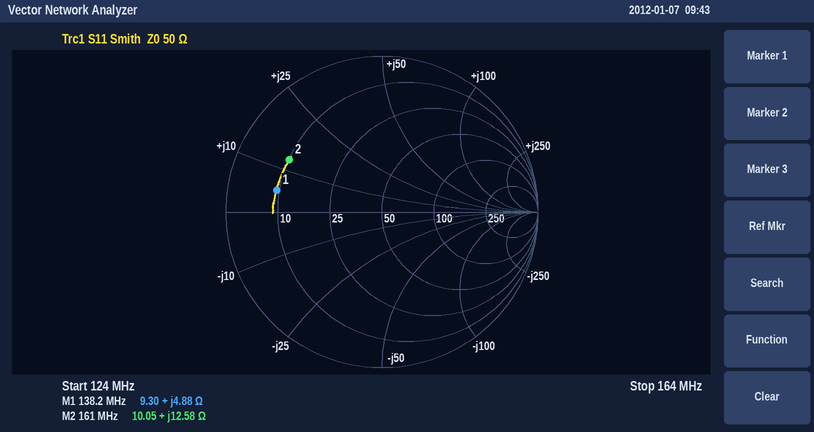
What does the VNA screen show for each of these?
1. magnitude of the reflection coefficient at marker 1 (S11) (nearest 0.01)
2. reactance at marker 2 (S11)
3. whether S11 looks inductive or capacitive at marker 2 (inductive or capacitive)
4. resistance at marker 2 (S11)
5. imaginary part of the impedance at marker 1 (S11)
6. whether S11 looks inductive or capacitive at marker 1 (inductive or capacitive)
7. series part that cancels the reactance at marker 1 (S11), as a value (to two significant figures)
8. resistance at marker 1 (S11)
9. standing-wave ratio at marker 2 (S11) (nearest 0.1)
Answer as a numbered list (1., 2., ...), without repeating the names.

1. 0.69
2. +12.58 Ω
3. inductive
4. 10.05 Ω
5. +4.88 Ω
6. inductive
7. 240 pF
8. 9.30 Ω
9. 5.3
